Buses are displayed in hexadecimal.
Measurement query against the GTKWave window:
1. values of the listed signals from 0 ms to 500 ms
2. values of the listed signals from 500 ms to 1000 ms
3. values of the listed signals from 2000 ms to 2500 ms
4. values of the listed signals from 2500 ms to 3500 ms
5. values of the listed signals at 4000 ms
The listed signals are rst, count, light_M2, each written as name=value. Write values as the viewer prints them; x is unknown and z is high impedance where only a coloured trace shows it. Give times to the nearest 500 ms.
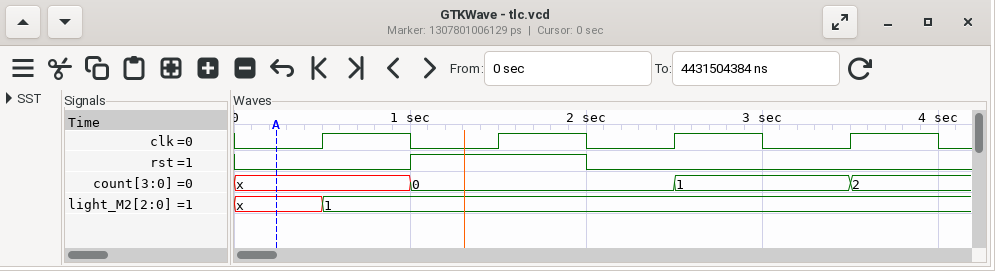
rst=0, count=x, light_M2=x
rst=0, count=x, light_M2=1
rst=0, count=0, light_M2=1
rst=0, count=1, light_M2=1
rst=0, count=2, light_M2=1
